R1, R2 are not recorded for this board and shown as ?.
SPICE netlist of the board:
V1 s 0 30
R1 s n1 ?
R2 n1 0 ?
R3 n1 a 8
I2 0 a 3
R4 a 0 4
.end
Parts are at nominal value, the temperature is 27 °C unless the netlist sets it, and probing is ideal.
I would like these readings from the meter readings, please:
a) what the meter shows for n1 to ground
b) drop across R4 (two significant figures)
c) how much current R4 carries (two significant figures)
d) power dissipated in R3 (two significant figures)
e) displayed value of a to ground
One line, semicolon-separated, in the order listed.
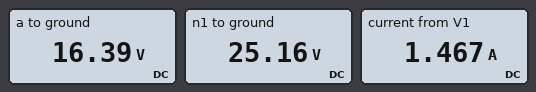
25.16 V; 16 V; 4.1 A; 9.6 W; 16.39 V
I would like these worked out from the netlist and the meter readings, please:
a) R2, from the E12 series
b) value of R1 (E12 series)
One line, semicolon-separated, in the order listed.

68 Ω; 3.3 Ω
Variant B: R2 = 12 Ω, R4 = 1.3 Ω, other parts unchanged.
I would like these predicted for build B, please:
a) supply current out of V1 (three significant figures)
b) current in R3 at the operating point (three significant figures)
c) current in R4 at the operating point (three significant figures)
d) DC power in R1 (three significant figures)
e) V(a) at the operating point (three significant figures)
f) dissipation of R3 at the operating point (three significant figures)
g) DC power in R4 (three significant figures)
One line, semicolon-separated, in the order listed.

3.26 A; 1.65 A; 4.65 A; 35.0 W; 6.05 V; 21.8 W; 28.1 W
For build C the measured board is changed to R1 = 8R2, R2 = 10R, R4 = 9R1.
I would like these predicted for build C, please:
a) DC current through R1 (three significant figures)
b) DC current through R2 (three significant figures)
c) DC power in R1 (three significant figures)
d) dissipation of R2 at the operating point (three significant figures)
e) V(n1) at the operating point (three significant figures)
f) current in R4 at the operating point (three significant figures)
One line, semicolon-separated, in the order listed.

1.37 A; 1.87 A; 15.5 W; 35.1 W; 18.7 V; 2.50 A
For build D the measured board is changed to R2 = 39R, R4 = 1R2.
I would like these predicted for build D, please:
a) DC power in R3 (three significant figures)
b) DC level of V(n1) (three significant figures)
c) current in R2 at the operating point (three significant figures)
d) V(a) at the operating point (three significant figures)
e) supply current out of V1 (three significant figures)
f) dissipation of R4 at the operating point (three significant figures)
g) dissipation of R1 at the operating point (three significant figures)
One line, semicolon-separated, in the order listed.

30.9 W; 21.7 V; 556 mA; 5.96 V; 2.52 A; 29.6 W; 21.0 W
